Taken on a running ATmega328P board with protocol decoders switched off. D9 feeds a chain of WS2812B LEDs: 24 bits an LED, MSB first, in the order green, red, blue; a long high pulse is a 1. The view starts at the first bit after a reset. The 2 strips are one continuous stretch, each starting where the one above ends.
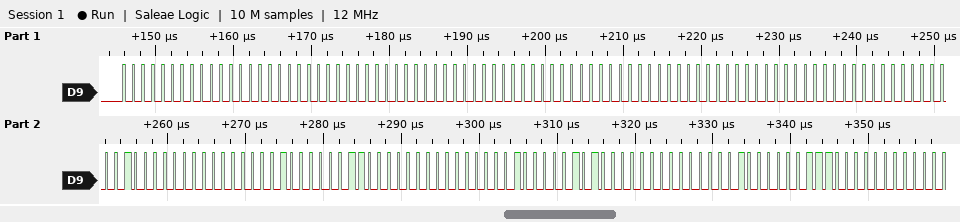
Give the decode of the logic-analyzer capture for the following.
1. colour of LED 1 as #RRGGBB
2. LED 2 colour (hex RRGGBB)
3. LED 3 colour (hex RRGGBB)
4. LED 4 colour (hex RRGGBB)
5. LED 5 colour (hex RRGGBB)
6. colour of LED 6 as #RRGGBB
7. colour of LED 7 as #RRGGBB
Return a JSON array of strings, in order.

["#000000", "#000000", "#000000", "#010000", "#030100", "#050100", "#070200"]
